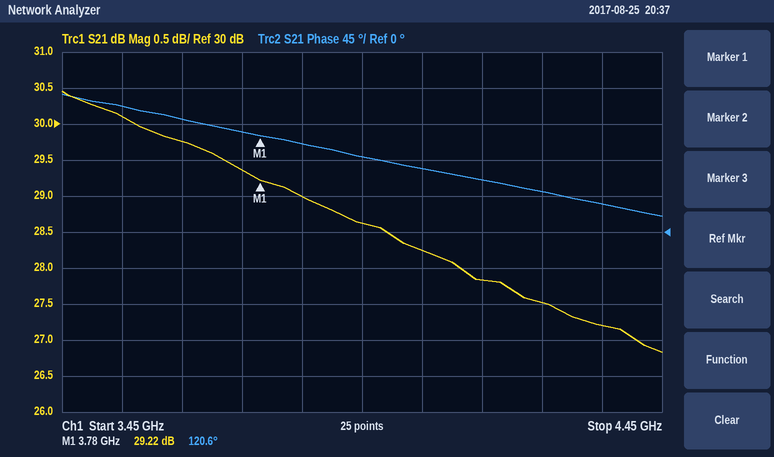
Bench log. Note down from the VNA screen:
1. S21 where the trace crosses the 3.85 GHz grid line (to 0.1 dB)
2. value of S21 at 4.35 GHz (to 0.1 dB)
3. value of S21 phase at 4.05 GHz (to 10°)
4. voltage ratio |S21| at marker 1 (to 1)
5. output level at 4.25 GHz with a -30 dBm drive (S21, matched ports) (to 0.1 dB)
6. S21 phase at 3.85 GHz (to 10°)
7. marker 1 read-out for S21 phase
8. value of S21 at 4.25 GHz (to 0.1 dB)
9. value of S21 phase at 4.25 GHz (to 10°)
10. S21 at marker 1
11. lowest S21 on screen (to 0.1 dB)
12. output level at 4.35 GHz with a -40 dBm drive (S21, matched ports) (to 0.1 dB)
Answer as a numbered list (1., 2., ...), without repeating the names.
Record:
1. 29.0 dB
2. 27.2 dB
3. 80°
4. 29
5. -2.5 dBm
6. 110°
7. 120.6°
8. 27.5 dB
9. 50°
10. 29.22 dB
11. 26.8 dB
12. -12.8 dBm
